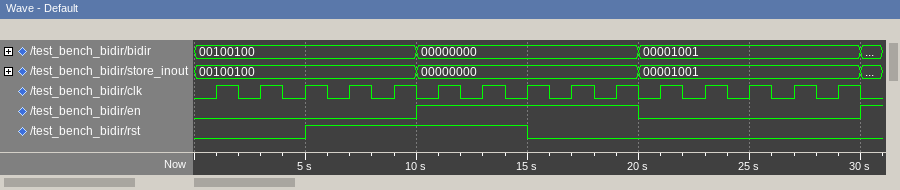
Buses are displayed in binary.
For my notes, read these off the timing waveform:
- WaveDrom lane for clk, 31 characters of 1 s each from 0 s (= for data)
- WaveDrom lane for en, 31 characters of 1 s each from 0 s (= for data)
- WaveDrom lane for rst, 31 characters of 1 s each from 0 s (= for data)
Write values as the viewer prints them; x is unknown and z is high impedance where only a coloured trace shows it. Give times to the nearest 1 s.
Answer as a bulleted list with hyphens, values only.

- {name: 'clk', wave: '0101010101010101010101010101010'}
- {name: 'en', wave: '0.........1.........0.........1'}
- {name: 'rst', wave: '0....1.........0...............'}
